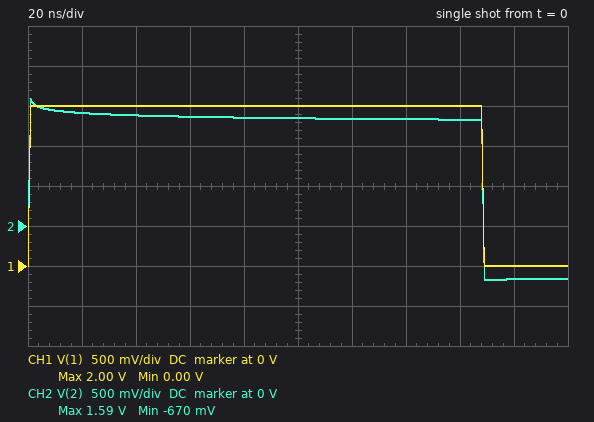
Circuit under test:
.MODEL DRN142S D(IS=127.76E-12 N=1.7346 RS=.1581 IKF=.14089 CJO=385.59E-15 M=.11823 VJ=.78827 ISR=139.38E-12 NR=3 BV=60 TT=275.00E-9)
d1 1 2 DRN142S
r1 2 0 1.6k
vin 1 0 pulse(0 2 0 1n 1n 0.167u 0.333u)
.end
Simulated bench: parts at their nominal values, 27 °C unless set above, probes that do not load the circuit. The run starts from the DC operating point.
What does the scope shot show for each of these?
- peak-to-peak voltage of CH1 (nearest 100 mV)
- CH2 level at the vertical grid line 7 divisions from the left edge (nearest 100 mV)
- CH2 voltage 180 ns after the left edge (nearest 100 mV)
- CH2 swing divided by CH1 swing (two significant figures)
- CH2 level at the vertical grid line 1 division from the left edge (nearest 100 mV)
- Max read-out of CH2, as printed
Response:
2.0 V
1.3 V
-700 mV
1.1
1.4 V
1.59 V
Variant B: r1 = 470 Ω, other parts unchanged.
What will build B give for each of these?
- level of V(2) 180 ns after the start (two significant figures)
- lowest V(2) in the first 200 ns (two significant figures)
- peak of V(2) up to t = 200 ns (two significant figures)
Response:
-720 mV
-730 mV
1.5 V
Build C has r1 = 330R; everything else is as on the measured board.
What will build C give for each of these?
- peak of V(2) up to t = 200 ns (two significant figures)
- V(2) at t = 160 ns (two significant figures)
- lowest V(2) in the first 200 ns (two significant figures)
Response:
1.5 V
1.3 V
-740 mV
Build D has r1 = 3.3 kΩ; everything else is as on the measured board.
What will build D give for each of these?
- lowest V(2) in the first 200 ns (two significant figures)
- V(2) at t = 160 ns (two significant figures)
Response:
-640 mV
1.4 V
